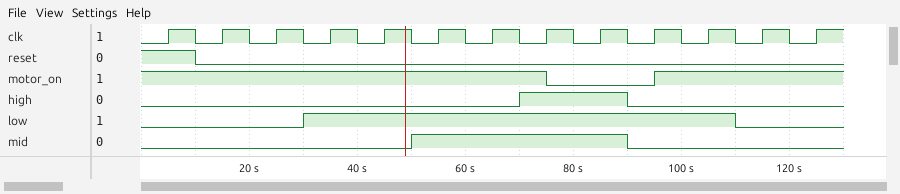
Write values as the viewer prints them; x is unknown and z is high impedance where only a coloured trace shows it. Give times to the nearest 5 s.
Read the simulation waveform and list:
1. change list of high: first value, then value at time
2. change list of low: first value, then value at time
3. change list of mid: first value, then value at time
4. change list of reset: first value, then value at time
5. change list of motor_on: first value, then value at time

0, 1 at 70 s, 0 at 90 s
0, 1 at 30 s, 0 at 110 s
0, 1 at 50 s, 0 at 90 s
1, 0 at 10 s
1, 0 at 75 s, 1 at 95 s
